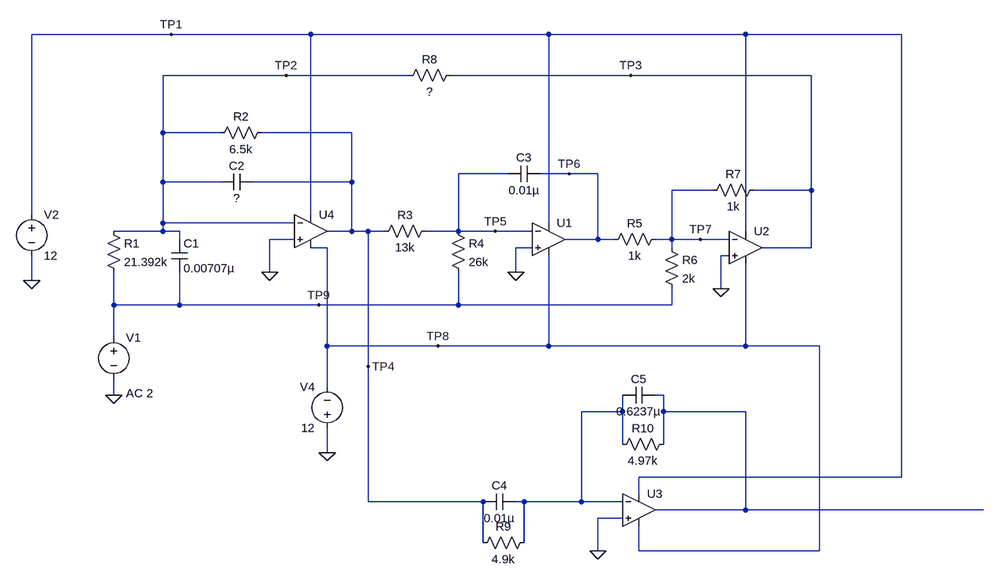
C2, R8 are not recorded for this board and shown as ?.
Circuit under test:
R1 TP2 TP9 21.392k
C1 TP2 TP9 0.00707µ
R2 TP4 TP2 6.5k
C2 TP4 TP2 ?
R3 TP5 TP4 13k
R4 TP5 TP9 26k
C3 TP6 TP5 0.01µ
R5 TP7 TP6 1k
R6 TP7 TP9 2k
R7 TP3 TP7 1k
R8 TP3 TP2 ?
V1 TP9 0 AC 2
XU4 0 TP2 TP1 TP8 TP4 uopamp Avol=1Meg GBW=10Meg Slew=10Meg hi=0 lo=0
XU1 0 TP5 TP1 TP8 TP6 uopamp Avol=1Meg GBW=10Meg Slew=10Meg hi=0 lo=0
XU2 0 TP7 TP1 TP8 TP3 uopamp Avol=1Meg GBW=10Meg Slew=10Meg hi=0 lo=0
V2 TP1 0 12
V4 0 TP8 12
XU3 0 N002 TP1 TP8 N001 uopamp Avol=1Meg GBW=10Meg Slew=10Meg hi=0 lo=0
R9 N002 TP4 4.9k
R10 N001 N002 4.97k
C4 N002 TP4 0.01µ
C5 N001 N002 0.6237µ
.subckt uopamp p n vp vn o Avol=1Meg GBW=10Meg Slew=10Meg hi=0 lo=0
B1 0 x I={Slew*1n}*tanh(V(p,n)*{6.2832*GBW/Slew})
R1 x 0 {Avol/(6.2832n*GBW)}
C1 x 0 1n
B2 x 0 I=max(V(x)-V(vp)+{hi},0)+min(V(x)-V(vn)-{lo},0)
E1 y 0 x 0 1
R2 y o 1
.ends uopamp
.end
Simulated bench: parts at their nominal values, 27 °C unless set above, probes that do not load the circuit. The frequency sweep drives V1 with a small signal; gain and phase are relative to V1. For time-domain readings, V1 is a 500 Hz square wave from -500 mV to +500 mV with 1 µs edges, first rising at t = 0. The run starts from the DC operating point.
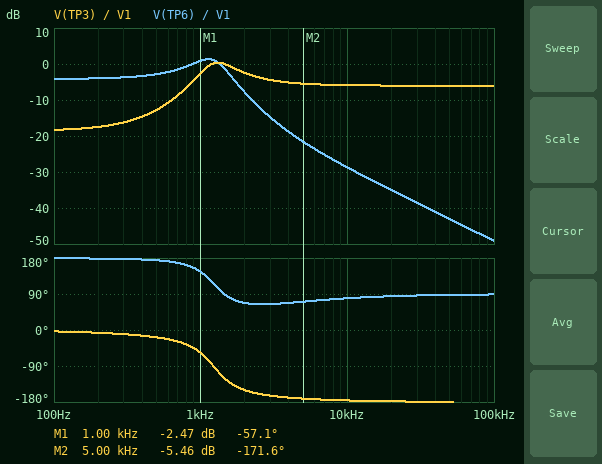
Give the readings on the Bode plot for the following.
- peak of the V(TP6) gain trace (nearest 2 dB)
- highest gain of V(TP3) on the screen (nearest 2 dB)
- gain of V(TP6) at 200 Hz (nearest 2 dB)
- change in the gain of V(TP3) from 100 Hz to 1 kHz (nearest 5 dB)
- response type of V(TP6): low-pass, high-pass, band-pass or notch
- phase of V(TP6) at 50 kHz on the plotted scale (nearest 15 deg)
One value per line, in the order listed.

2 dB
0 dB
-4 dB
15 dB
low-pass
90 deg
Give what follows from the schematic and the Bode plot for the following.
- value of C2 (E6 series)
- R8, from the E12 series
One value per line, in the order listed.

33 nF
3.9 kΩ
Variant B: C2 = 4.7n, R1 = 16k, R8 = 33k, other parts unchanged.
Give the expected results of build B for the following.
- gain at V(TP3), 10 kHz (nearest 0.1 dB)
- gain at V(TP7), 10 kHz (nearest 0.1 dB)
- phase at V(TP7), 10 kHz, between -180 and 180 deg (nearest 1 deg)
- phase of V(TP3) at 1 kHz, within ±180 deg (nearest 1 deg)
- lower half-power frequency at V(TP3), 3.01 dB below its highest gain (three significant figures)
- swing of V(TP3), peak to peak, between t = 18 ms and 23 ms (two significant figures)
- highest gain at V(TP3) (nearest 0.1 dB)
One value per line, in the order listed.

-4.9 dB
-64.9 dB
80 deg
-161 deg
114 Hz
1.4 V
-2.3 dB
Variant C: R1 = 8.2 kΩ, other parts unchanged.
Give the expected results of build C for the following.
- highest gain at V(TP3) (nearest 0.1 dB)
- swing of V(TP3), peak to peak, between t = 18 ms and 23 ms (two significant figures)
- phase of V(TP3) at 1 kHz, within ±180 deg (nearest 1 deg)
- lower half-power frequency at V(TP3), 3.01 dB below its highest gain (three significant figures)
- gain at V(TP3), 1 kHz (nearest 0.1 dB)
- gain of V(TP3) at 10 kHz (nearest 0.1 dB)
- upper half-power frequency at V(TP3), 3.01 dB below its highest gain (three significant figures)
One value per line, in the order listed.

-3.8 dB
820 mV
-60 deg
1.15 kHz
-11.7 dB
-6.0 dB
1.80 MHz
